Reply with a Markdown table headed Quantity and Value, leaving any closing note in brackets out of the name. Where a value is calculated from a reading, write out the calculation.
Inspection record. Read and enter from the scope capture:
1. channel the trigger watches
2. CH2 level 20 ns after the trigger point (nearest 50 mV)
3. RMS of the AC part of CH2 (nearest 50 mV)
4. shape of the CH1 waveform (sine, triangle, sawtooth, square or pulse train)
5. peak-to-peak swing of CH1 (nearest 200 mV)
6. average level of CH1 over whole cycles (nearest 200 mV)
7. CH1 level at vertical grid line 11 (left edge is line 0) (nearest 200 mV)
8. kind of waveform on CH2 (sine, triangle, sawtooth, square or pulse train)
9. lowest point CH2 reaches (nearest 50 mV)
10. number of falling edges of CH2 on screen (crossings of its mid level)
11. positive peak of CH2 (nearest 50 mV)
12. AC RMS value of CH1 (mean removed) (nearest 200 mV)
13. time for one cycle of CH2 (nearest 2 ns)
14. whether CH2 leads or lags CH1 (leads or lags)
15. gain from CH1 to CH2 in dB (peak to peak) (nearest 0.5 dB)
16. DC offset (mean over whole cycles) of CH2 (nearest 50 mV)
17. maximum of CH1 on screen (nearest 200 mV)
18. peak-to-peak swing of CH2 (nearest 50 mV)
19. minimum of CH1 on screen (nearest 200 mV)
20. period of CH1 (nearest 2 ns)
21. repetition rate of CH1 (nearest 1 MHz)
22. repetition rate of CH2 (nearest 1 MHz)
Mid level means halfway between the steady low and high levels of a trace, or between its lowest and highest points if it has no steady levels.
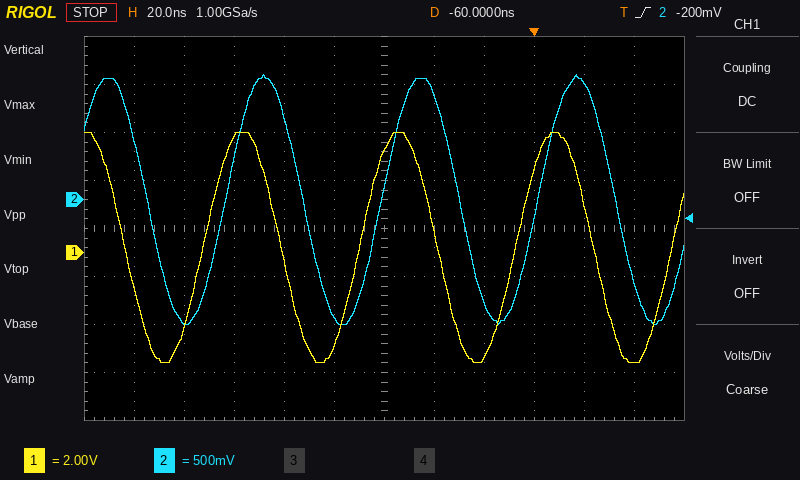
| Quantity | Value |
|---|---|
| channel the trigger watches | CH2 |
| CH2 level 20 ns after the trigger point | 1.20 V |
| RMS of the AC part of CH2 | 2.60 V / (2√2) ≈ 919 mV, so 900 mV to the nearest 50 mV |
| shape of the CH1 waveform | sine |
| peak-to-peak swing of CH1 | 5.0 V − (-4.6 V) = 9.6 V |
| average level of CH1 over whole cycles | (5.0 V + (-4.6 V)) / 2 ≈ 200 mV |
| CH1 level at vertical grid line 11 (left edge is line 0) | -4.6 V |
| kind of waveform on CH2 | sine |
| lowest point CH2 reaches | -1.30 V |
| number of falling edges of CH2 on screen | 4 |
| positive peak of CH2 | 1.30 V |
| AC RMS value of CH1 (mean removed) | 9.6 V / (2√2) ≈ 3.4 V |
| time for one cycle of CH2 | 62 ns |
| whether CH2 leads or lags CH1 | lags |
| gain from CH1 to CH2 in dB (peak to peak) | 20 log10(2.60 V / 9.6 V) ≈ -11.3 dB, so -11.5 dB to the nearest 0.5 dB |
| DC offset (mean over whole cycles) of CH2 | (1.30 V + (-1.30 V)) / 2 ≈ 0 mV |
| maximum of CH1 on screen | 5.0 V |
| peak-to-peak swing of CH2 | 1.30 V − (-1.30 V) = 2.60 V |
| minimum of CH1 on screen | -4.6 V |
| period of CH1 | 62 ns |
| repetition rate of CH1 | 1 / 62 ns ≈ 16 MHz |
| repetition rate of CH2 | 1 / 62 ns ≈ 16 MHz |
